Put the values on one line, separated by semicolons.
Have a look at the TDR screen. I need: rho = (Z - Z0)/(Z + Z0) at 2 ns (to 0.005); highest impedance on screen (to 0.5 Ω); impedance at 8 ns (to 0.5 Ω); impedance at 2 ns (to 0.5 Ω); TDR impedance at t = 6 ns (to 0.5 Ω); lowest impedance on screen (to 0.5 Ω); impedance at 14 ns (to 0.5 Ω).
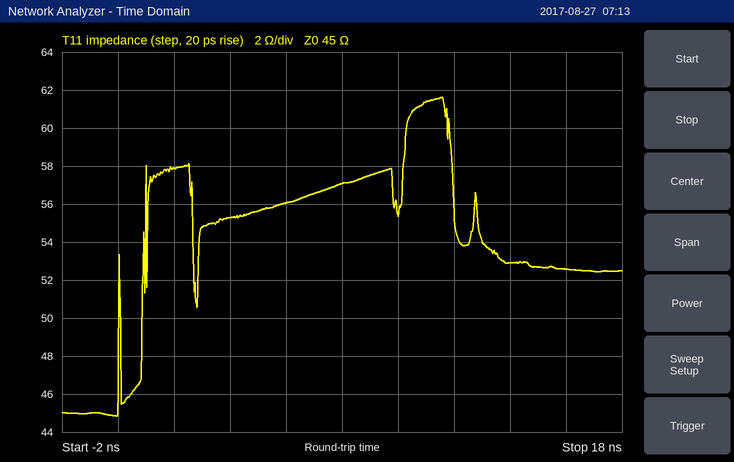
+0.125; 61.5 Ω; 57.0 Ω; 58.0 Ω; 56.0 Ω; 45.0 Ω; 53.0 Ω
